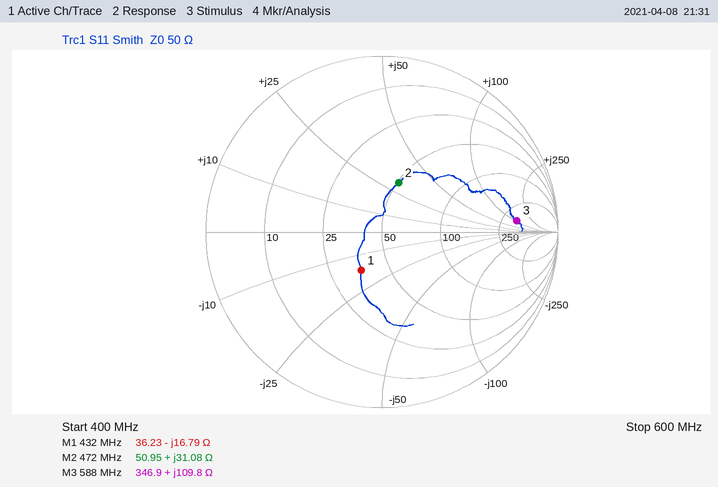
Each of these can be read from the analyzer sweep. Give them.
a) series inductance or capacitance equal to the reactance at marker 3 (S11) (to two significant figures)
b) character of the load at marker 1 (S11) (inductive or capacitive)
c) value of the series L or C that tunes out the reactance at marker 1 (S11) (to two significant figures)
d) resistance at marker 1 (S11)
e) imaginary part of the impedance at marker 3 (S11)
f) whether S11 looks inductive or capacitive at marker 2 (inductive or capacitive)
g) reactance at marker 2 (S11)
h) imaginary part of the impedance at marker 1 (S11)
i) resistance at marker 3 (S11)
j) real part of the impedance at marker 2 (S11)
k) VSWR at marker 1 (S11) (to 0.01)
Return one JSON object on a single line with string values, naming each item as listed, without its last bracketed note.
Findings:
{"series inductance or capacitance equal to the reactance at marker 3 (S11)": "30 nH", "character of the load at marker 1 (S11)": "capacitive", "value of the series L or C that tunes out the reactance at marker 1 (S11)": "6.2 nH", "resistance at marker 1": "36.23 Ω", "imaginary part of the impedance at marker 3": "+109.8 Ω", "whether S11 looks inductive or capacitive at marker 2": "inductive", "reactance at marker 2": "+31.08 Ω", "imaginary part of the impedance at marker 1": "-16.79 Ω", "resistance at marker 3": "346.9 Ω", "real part of the impedance at marker 2": "50.95 Ω", "VSWR at marker 1 (S11)": "1.66"}
